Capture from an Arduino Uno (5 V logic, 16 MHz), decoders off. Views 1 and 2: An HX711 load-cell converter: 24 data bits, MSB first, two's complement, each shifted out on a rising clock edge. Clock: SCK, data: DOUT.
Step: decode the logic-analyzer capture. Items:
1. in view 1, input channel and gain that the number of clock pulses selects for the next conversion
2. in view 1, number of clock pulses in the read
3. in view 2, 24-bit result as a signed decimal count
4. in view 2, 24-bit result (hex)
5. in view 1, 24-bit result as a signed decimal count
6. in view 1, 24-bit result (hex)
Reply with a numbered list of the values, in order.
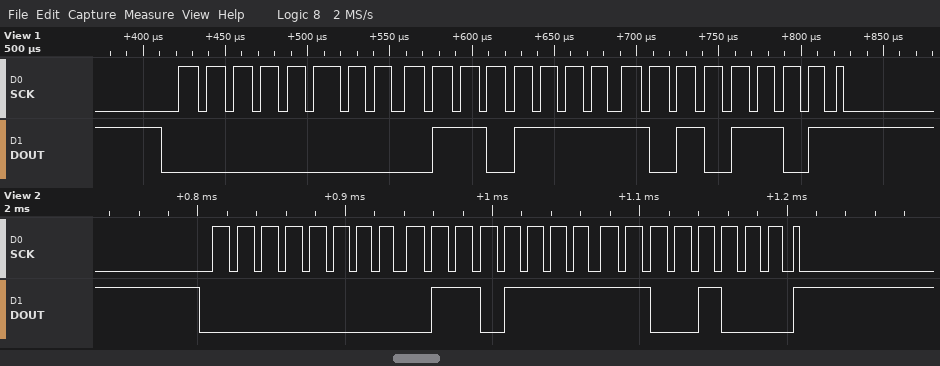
1. channel A, gain 128
2. 25
3. 28616
4. 0x006FC8
5. 28589
6. 0x006FAD
